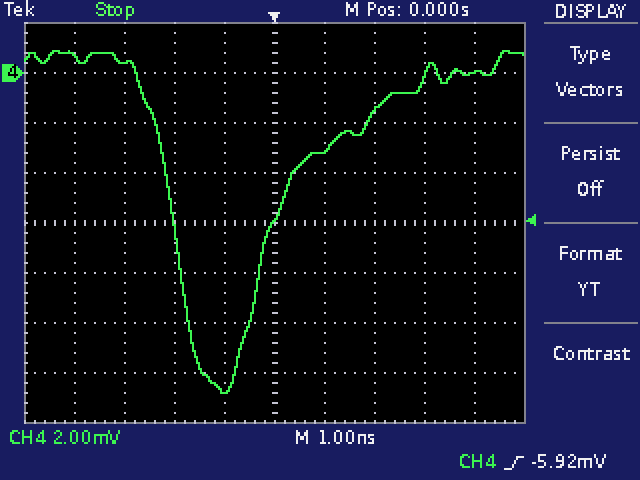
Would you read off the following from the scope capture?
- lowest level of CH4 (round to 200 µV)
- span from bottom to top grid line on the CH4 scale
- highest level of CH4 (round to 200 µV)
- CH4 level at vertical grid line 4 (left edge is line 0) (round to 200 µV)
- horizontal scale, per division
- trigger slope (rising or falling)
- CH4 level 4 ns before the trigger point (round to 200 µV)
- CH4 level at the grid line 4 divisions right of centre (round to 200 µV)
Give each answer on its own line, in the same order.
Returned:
-12.8 mV
16 mV
800 µV
-12.8 mV
1 ns
rising
600 µV
0.0 mV
